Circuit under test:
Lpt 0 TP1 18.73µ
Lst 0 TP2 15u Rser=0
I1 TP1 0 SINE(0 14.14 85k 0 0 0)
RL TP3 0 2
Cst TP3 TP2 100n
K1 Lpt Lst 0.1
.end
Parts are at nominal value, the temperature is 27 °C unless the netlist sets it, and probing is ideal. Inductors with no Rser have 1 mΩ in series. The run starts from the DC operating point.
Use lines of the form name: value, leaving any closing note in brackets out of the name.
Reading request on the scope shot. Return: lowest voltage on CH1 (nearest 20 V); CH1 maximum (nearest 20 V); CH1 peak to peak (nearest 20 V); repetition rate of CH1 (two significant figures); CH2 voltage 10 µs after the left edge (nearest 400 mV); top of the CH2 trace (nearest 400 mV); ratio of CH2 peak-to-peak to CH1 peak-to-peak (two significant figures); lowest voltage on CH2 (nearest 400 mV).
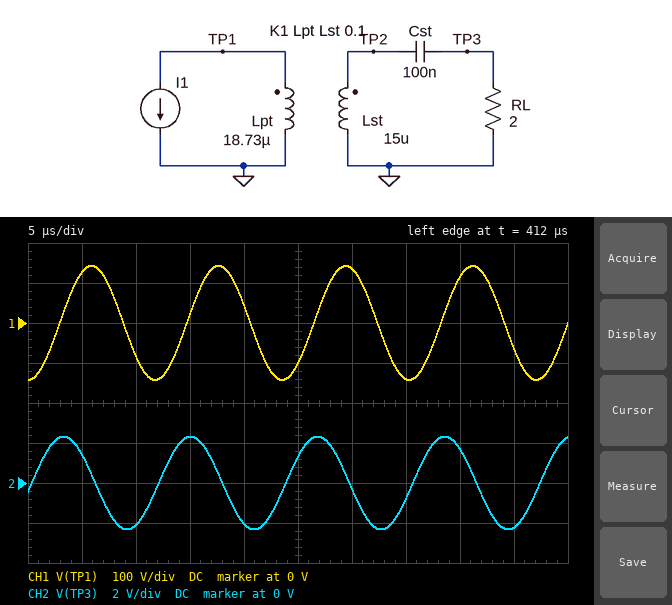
lowest voltage on CH1: -140 V
CH1 maximum: 140 V
CH1 peak to peak: 280 V
repetition rate of CH1: 85 kHz
CH2 voltage 10 µs after the left edge: -2.0 V
top of the CH2 trace: 2.4 V
ratio of CH2 peak-to-peak to CH1 peak-to-peak: 0.016
lowest voltage on CH2: -2.4 V
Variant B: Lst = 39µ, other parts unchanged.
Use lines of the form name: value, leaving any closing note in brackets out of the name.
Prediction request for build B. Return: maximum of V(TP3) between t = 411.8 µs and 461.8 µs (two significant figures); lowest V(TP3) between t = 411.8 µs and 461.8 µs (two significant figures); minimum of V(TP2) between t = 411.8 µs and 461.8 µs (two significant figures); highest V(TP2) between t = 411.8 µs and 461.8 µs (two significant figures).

maximum of V(TP3) between t = 411.8 µs and 461.8 µs: 14 V
lowest V(TP3) between t = 411.8 µs and 461.8 µs: -14 V
minimum of V(TP2) between t = 411.8 µs and 461.8 µs: -130 V
highest V(TP2) between t = 411.8 µs and 461.8 µs: 130 V
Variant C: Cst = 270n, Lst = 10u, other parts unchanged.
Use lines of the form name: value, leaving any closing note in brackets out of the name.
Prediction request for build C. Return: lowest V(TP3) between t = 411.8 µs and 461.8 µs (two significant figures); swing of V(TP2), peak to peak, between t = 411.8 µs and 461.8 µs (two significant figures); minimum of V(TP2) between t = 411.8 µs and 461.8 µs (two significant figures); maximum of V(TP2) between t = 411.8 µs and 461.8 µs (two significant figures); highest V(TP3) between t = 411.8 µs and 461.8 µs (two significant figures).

lowest V(TP3) between t = 411.8 µs and 461.8 µs: -8.1 V
swing of V(TP2), peak to peak, between t = 411.8 µs and 461.8 µs: 58 V
minimum of V(TP2) between t = 411.8 µs and 461.8 µs: -29 V
maximum of V(TP2) between t = 411.8 µs and 461.8 µs: 29 V
highest V(TP3) between t = 411.8 µs and 461.8 µs: 8.1 V
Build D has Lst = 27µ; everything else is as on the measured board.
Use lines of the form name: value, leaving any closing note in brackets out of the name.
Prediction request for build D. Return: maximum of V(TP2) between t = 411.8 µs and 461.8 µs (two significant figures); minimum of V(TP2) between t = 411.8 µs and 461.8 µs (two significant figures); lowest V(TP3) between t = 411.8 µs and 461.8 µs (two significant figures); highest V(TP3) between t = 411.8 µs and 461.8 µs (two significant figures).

maximum of V(TP2) between t = 411.8 µs and 461.8 µs: 67 V
minimum of V(TP2) between t = 411.8 µs and 461.8 µs: -67 V
lowest V(TP3) between t = 411.8 µs and 461.8 µs: -7.2 V
highest V(TP3) between t = 411.8 µs and 461.8 µs: 7.2 V
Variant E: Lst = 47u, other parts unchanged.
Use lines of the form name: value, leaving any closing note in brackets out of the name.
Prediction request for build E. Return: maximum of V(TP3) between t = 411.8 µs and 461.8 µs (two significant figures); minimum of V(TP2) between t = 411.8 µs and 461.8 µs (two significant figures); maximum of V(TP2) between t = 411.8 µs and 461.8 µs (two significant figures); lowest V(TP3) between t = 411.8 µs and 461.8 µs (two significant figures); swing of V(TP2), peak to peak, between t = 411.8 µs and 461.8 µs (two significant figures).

maximum of V(TP3) between t = 411.8 µs and 461.8 µs: 6.7 V
minimum of V(TP2) between t = 411.8 µs and 461.8 µs: -63 V
maximum of V(TP2) between t = 411.8 µs and 461.8 µs: 63 V
lowest V(TP3) between t = 411.8 µs and 461.8 µs: -6.7 V
swing of V(TP2), peak to peak, between t = 411.8 µs and 461.8 µs: 130 V
